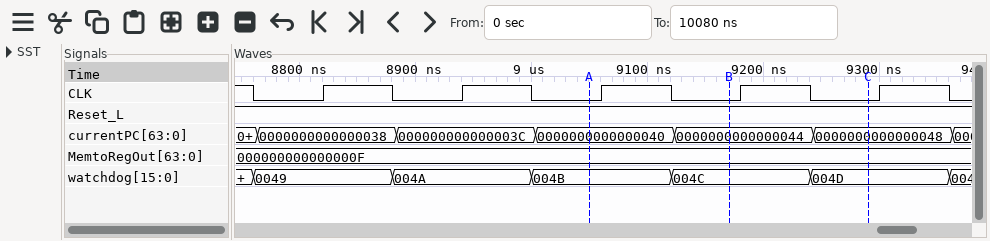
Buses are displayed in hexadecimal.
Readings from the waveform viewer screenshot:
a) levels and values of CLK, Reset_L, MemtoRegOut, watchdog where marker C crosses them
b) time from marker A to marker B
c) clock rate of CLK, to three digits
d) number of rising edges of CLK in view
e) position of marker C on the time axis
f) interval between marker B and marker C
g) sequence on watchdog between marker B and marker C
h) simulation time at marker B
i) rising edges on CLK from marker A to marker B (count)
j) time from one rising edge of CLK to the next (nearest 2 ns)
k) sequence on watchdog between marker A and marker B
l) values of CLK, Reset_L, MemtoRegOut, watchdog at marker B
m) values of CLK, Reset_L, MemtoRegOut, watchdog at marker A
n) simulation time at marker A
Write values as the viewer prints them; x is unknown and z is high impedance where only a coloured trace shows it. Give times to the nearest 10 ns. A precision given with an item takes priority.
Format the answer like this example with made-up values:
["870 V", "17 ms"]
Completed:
["CLK=0, Reset_L=1, MemtoRegOut=000000000000000F, watchdog=004D", "120 ns", "8.33 MHz", "5", "9290 ns", "120 ns", "004C, 004D", "9170 ns", "1", "120 ns", "004B, 004C", "CLK=0, Reset_L=1, MemtoRegOut=000000000000000F, watchdog=004C", "CLK=0, Reset_L=1, MemtoRegOut=000000000000000F, watchdog=004B", "9050 ns"]
